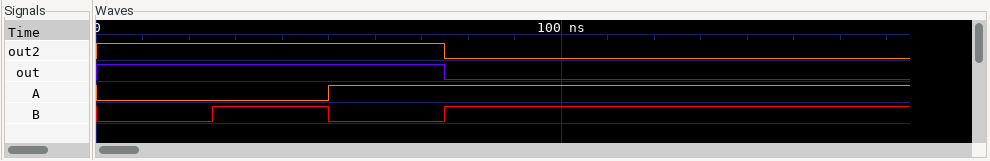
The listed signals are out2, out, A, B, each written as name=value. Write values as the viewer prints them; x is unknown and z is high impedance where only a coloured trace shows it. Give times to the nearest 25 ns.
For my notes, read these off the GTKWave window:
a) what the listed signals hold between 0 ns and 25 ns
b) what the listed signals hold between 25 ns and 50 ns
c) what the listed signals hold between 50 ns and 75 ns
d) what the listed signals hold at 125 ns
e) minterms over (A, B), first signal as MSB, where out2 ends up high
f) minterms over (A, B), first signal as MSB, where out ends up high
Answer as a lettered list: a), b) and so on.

a) out2=1, out=1, A=0, B=0
b) out2=1, out=1, A=0, B=1
c) out2=1, out=1, A=1, B=0
d) out2=0, out=0, A=1, B=1
e) 0, 1, 2
f) 0, 1, 2
